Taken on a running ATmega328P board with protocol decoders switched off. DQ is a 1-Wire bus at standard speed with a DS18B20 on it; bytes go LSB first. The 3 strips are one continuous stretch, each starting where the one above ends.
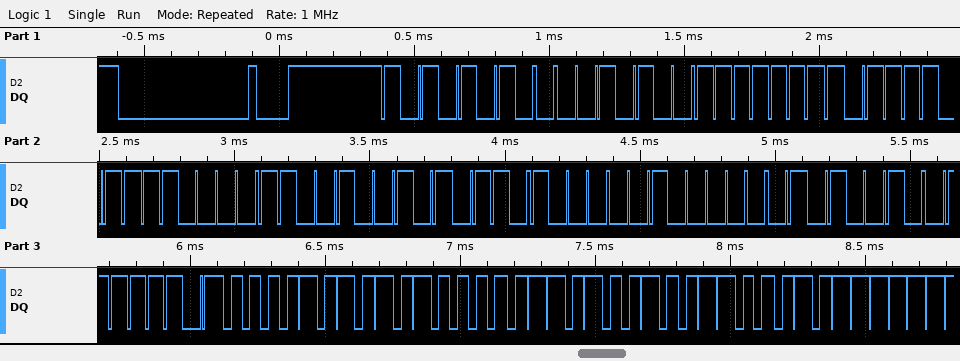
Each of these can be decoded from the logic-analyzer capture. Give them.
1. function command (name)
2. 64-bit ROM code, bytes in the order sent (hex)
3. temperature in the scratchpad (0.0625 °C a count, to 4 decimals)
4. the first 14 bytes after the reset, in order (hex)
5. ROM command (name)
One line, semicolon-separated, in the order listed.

Read Scratchpad; 28 FF DE C3 A4 16 04 4A; 85.0000 °C; 55 28 FF DE C3 A4 16 04 4A BE 50 05 4B 46; Match ROM
